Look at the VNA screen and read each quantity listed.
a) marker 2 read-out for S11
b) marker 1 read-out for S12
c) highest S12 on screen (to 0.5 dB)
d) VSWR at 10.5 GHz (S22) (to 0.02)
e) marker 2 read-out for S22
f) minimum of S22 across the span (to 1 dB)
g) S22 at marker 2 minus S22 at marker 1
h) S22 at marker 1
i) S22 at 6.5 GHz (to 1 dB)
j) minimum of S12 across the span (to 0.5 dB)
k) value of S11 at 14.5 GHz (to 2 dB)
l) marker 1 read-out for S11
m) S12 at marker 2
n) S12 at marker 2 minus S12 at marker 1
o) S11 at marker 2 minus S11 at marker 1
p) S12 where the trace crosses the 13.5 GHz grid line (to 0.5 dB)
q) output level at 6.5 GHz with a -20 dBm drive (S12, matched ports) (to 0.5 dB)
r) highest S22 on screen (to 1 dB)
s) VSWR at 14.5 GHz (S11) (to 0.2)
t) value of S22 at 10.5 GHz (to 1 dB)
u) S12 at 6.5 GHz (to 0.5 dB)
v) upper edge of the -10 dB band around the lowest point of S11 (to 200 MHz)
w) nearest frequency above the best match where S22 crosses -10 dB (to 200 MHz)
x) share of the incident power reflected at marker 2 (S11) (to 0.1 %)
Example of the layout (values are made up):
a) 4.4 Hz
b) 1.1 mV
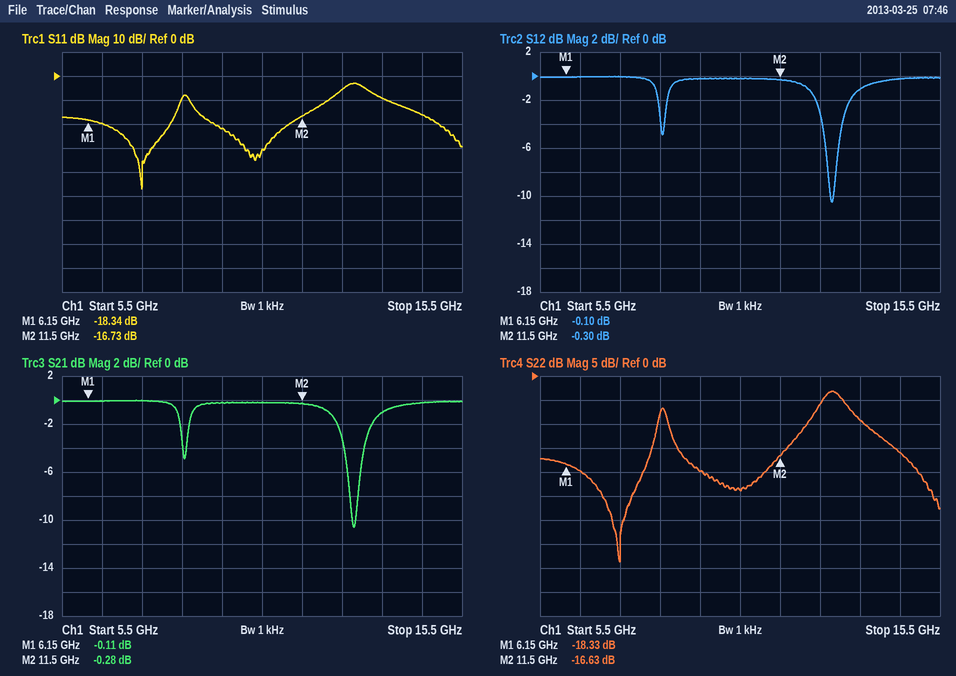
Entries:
a) -16.73 dB
b) -0.10 dB
c) 0.0 dB
d) 1.14
e) -16.63 dB
f) -39 dB
g) 1.70 dB
h) -18.33 dB
i) -20 dB
j) -10.5 dB
k) -16 dB
l) -18.34 dB
m) -0.30 dB
n) -0.20 dB
o) 1.61 dB
p) -1.0 dB
q) -20.0 dBm
r) -3 dB
s) 1.4
t) -24 dB
u) 0.0 dB
v) 8.4 GHz
w) 8.4 GHz
x) 2.1 %
